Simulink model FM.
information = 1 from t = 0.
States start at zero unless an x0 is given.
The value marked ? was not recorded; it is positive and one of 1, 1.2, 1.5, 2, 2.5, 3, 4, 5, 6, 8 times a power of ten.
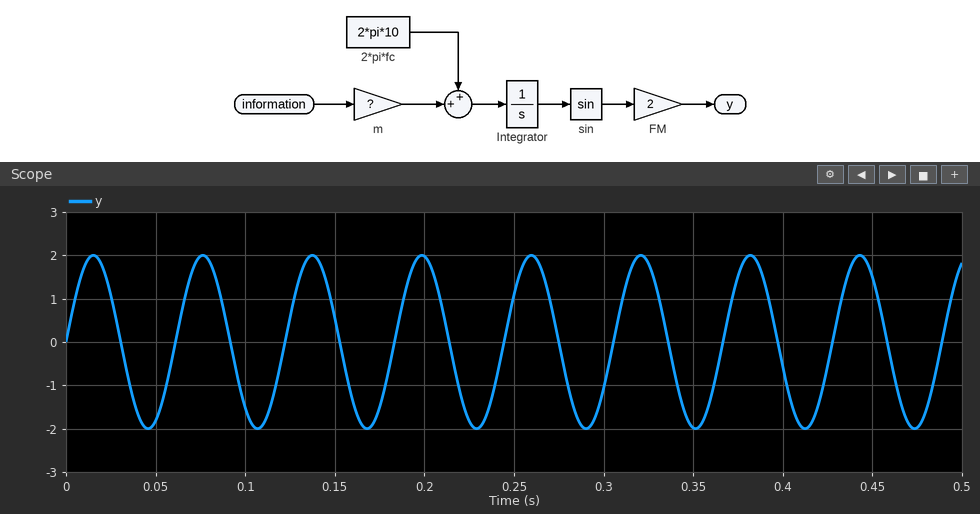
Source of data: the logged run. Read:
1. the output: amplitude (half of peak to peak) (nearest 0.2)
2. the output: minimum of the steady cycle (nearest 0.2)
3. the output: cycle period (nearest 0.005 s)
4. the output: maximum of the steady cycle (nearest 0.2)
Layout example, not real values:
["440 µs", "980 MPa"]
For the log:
["2.0", "-2.0", "0.060 s", "2.0"]
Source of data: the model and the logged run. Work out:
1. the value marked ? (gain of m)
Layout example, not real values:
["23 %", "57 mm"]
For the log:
["40"]
